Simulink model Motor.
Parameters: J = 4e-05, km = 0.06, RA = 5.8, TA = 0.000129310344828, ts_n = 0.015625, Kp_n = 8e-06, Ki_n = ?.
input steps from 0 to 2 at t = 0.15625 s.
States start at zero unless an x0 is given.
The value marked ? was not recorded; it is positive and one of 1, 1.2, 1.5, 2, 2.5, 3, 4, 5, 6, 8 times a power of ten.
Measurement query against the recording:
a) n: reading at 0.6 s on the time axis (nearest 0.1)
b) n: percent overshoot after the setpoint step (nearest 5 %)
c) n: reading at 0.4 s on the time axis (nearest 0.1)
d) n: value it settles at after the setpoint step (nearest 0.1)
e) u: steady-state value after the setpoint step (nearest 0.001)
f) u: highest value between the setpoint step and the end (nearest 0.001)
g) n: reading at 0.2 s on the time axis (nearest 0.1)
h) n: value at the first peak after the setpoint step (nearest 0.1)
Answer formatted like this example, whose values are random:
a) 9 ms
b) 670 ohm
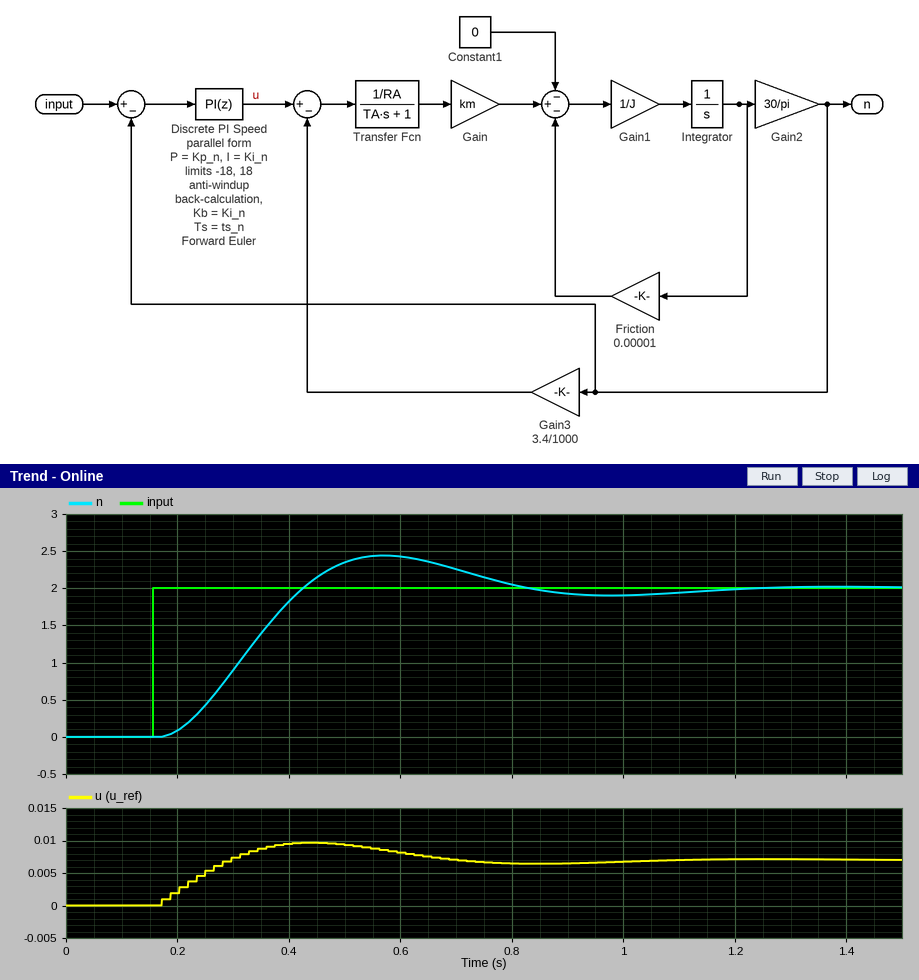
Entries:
a) 2.4
b) 20 %
c) 1.8
d) 2.0
e) 0.007
f) 0.010
g) 0.1
h) 2.4
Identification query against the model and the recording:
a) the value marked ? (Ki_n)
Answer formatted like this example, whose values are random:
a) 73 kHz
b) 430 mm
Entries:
a) 0.03
